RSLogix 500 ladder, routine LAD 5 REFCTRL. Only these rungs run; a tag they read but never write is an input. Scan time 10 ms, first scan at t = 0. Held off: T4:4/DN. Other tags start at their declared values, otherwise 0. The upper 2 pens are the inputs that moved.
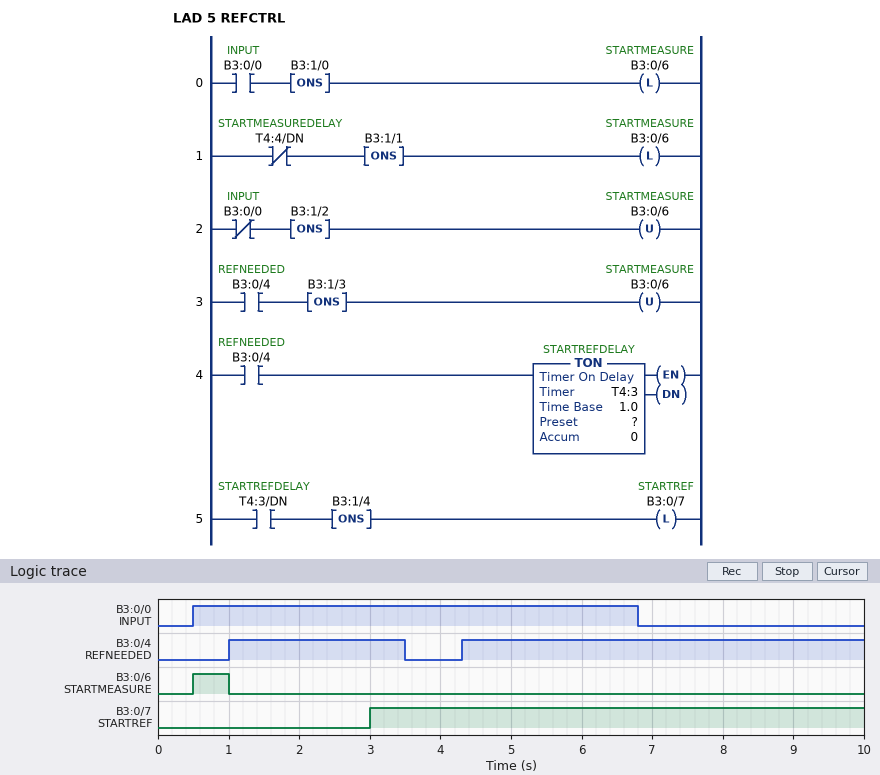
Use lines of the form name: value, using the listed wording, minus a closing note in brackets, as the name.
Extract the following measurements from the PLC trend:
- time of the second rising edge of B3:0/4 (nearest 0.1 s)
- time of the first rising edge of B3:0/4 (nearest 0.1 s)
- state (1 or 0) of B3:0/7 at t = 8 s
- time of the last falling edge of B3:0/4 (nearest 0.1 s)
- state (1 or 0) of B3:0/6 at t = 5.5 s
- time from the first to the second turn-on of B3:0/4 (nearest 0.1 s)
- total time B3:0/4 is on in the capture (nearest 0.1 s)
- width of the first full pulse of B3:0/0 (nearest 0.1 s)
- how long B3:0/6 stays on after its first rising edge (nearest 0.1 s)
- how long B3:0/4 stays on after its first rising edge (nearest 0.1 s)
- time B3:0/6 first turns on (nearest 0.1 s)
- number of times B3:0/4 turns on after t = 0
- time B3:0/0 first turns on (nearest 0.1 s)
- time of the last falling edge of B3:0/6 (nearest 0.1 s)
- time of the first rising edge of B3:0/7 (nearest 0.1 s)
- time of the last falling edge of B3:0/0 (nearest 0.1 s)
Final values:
time of the second rising edge of B3:0/4: 4.3 s
time of the first rising edge of B3:0/4: 1.0 s
state (1 or 0) of B3:0/7 at t = 8 s: 1
time of the last falling edge of B3:0/4: 3.5 s
state (1 or 0) of B3:0/6 at t = 5.5 s: 0
time from the first to the second turn-on of B3:0/4: 3.3 s
total time B3:0/4 is on in the capture: 8.2 s
width of the first full pulse of B3:0/0: 6.3 s
how long B3:0/6 stays on after its first rising edge: 0.5 s
how long B3:0/4 stays on after its first rising edge: 2.5 s
time B3:0/6 first turns on: 0.5 s
number of times B3:0/4 turns on after t = 0: 2
time B3:0/0 first turns on: 0.5 s
time of the last falling edge of B3:0/6: 1.0 s
time of the first rising edge of B3:0/7: 3.0 s
time of the last falling edge of B3:0/0: 6.8 s
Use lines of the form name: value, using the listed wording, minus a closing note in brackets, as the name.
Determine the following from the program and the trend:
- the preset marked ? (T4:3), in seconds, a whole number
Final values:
the preset marked ? (T4:3), in seconds, a whole number: 2 s
